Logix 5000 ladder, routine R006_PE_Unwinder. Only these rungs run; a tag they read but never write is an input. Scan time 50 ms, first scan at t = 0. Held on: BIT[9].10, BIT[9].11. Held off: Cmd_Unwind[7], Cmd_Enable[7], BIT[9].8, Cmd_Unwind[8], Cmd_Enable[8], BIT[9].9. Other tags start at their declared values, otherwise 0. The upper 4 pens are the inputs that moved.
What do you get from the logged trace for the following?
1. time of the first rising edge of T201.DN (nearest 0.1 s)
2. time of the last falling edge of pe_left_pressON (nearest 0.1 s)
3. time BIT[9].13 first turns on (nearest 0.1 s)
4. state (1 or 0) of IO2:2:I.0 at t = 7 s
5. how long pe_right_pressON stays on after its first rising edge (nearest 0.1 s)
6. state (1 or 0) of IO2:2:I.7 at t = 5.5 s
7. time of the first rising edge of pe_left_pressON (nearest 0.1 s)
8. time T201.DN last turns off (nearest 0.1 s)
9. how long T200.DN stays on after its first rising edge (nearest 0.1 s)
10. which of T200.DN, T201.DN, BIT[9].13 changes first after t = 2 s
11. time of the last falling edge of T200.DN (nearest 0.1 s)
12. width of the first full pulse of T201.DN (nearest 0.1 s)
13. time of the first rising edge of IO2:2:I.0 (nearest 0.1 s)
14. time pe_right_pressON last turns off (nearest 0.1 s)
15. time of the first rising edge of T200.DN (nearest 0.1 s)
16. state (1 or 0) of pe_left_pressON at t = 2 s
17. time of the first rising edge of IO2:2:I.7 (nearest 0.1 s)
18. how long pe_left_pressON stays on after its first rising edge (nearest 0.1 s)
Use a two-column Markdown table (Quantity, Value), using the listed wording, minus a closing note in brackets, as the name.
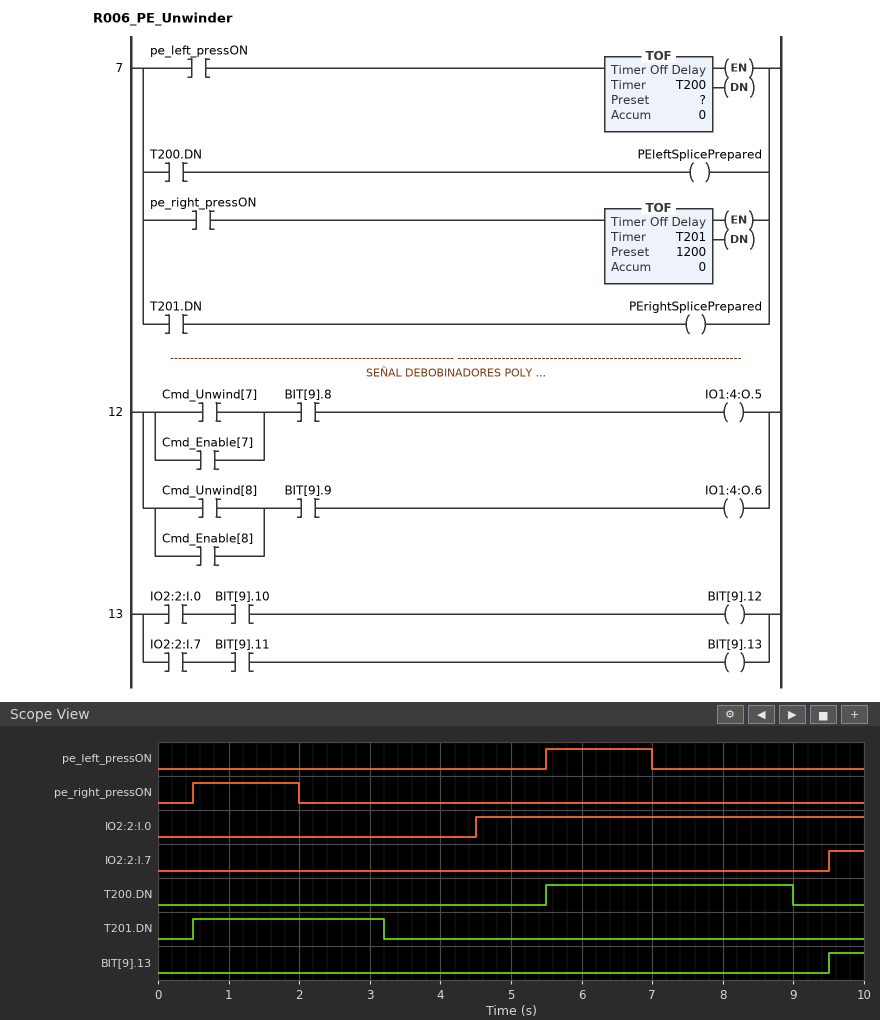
| Quantity | Value |
|---|---|
| time of the first rising edge of T201.DN | 0.5 s |
| time of the last falling edge of pe_left_pressON | 7.0 s |
| time BIT[9].13 first turns on | 9.5 s |
| state (1 or 0) of IO2:2:I.0 at t = 7 s | 1 |
| how long pe_right_pressON stays on after its first rising edge | 1.5 s |
| state (1 or 0) of IO2:2:I.7 at t = 5.5 s | 0 |
| time of the first rising edge of pe_left_pressON | 5.5 s |
| time T201.DN last turns off | 3.2 s |
| how long T200.DN stays on after its first rising edge | 3.5 s |
| which of T200.DN, T201.DN, BIT[9].13 changes first after t = 2 s | T201.DN |
| time of the last falling edge of T200.DN | 9.0 s |
| width of the first full pulse of T201.DN | 2.7 s |
| time of the first rising edge of IO2:2:I.0 | 4.5 s |
| time pe_right_pressON last turns off | 2.0 s |
| time of the first rising edge of T200.DN | 5.5 s |
| state (1 or 0) of pe_left_pressON at t = 2 s | 0 |
| time of the first rising edge of IO2:2:I.7 | 9.5 s |
| how long pe_left_pressON stays on after its first rising edge | 1.5 s |
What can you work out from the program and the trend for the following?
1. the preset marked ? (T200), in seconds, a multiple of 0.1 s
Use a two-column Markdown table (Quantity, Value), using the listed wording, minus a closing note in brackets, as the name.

| Quantity | Value |
|---|---|
| the preset marked ? (T200), in seconds, a multiple of 0.1 s | 2.0 s |
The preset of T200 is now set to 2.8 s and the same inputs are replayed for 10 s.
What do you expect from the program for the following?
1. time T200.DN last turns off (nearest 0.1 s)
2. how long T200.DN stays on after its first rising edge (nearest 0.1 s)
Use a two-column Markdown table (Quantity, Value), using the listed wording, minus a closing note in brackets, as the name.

| Quantity | Value |
|---|---|
| time T200.DN last turns off | 9.8 s |
| how long T200.DN stays on after its first rising edge | 4.3 s |
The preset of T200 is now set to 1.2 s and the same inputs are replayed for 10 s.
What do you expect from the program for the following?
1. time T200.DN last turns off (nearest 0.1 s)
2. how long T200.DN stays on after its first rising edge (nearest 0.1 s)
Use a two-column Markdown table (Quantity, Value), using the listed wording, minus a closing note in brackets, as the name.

| Quantity | Value |
|---|---|
| time T200.DN last turns off | 8.2 s |
| how long T200.DN stays on after its first rising edge | 2.7 s |
